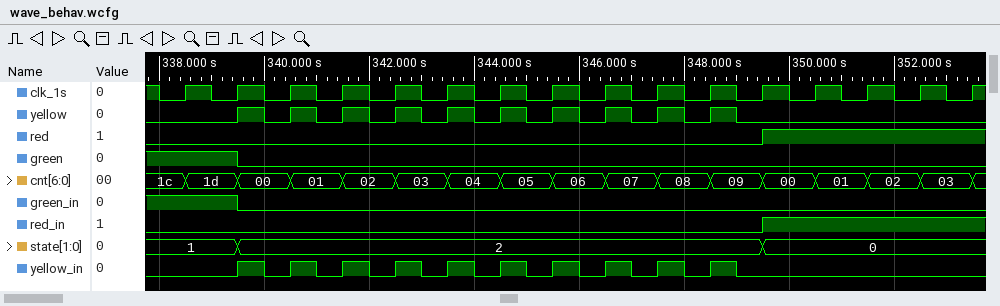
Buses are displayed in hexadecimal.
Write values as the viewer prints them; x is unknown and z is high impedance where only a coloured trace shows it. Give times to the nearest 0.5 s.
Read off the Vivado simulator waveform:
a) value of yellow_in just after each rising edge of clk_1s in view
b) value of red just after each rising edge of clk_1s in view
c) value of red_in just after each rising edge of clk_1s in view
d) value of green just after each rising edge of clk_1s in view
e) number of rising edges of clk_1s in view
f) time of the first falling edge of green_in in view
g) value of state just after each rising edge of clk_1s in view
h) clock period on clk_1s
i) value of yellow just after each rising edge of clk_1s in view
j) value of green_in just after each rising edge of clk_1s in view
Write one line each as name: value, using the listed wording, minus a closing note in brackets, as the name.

value of yellow_in just after each rising edge of clk_1s in view: 0 1 1 1 1 1 1 1 1 1 1 0 0 0 0 0
value of red just after each rising edge of clk_1s in view: 0 0 0 0 0 0 0 0 0 0 0 1 1 1 1 1
value of red_in just after each rising edge of clk_1s in view: 0 0 0 0 0 0 0 0 0 0 0 1 1 1 1 1
value of green just after each rising edge of clk_1s in view: 1 0 0 0 0 0 0 0 0 0 0 0 0 0 0 0
number of rising edges of clk_1s in view: 16
time of the first falling edge of green_in in view: 339.5 s
value of state just after each rising edge of clk_1s in view: 1, 2, 2, 2, 2, 2, 2, 2, 2, 2, 2, 0, 0, 0, 0, 0
clock period on clk_1s: 1 s
value of yellow just after each rising edge of clk_1s in view: 0 1 1 1 1 1 1 1 1 1 1 0 0 0 0 0
value of green_in just after each rising edge of clk_1s in view: 1 0 0 0 0 0 0 0 0 0 0 0 0 0 0 0
